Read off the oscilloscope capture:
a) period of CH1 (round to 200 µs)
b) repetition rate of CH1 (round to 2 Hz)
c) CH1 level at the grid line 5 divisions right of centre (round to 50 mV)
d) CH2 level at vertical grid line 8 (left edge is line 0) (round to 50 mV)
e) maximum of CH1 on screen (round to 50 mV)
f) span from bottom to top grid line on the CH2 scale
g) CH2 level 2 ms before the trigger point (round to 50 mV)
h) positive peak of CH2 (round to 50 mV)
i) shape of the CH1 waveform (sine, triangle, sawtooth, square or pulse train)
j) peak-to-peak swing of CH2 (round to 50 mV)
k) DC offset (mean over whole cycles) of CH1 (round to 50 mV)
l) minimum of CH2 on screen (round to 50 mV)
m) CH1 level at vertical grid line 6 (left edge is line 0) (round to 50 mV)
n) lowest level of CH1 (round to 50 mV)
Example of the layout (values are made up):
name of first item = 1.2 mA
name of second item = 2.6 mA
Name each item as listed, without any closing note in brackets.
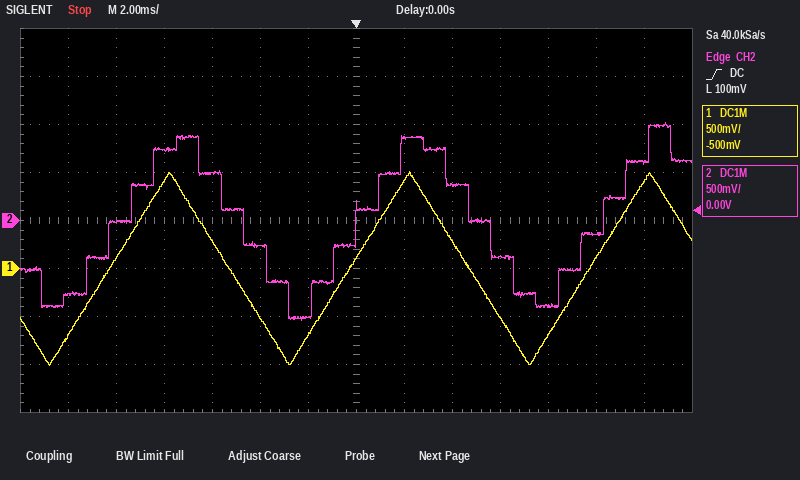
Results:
period of CH1 = 10.0 ms
repetition rate of CH1 = 100 Hz
CH1 level at the grid line 5 divisions right of centre = 100 mV
CH2 level at vertical grid line 8 (left edge is line 0) = 850 mV
maximum of CH1 on screen = 1.00 V
span from bottom to top grid line on the CH2 scale = 4 V
CH2 level 2 ms before the trigger point = -1.00 V
positive peak of CH2 = 1.00 V
shape of the CH1 waveform = triangle
peak-to-peak swing of CH2 = 2.05 V
DC offset (mean over whole cycles) of CH1 = 0 mV
minimum of CH2 on screen = -1.05 V
CH1 level at vertical grid line 6 (left edge is line 0) = -700 mV
lowest level of CH1 = -1.00 V
